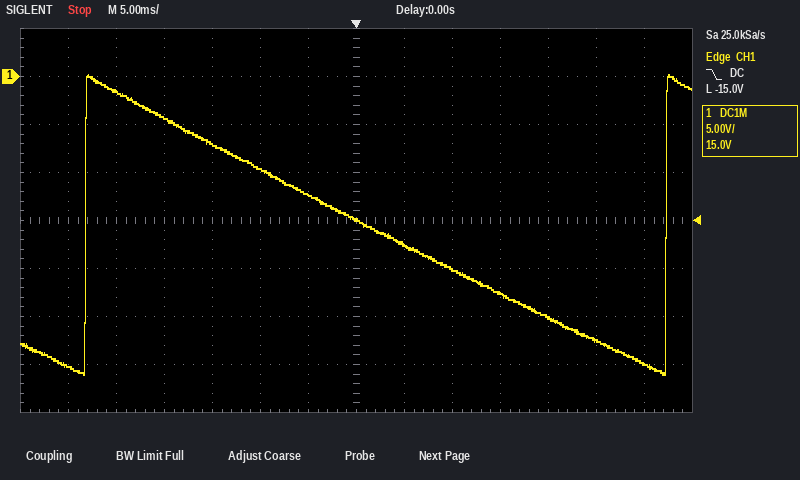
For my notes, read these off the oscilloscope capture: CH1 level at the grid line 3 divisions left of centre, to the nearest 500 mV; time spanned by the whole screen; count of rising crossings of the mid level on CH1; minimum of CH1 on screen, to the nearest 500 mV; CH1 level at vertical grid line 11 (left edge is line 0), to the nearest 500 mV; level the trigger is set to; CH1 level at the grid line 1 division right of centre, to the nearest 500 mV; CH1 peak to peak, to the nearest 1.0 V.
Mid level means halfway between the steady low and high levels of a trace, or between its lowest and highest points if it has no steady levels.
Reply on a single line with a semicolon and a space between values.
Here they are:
-7.0 V; 70 ms; 2; -31.0 V; -25.0 V; -15.0 V; -17.5 V; 31.0 V
